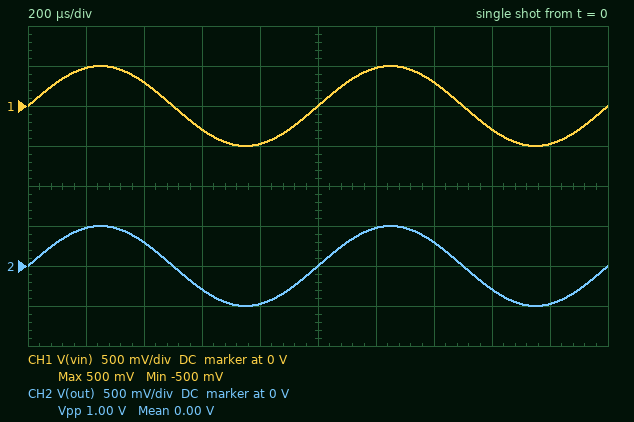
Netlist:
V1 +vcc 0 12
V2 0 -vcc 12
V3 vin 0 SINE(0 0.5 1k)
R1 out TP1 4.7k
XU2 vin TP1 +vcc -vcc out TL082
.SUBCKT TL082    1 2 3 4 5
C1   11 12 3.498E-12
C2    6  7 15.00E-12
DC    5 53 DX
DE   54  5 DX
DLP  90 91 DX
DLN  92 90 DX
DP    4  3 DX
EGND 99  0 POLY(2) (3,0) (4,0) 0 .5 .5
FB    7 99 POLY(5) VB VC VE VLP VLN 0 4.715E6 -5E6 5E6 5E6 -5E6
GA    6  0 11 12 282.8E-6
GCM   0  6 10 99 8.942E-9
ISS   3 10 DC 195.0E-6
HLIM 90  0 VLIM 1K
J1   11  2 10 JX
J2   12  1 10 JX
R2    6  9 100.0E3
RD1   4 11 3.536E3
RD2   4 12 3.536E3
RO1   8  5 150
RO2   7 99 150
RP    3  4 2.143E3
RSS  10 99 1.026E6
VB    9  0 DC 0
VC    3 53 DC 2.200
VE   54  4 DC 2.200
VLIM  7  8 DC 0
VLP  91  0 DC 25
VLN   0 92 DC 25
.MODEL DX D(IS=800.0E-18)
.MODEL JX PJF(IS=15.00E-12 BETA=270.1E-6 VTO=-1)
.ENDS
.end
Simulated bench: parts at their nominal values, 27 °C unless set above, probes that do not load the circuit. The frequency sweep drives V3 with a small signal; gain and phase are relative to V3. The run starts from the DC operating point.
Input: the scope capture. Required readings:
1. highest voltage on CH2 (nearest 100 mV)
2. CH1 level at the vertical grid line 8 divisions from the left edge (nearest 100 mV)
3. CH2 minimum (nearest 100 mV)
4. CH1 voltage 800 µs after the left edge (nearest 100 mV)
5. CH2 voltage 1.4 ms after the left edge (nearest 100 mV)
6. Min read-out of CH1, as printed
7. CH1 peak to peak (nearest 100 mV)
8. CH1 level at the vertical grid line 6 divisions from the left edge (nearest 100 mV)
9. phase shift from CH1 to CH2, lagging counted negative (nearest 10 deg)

500 mV
-300 mV
-500 mV
-500 mV
300 mV
-500 mV
1.0 V
500 mV
0 deg
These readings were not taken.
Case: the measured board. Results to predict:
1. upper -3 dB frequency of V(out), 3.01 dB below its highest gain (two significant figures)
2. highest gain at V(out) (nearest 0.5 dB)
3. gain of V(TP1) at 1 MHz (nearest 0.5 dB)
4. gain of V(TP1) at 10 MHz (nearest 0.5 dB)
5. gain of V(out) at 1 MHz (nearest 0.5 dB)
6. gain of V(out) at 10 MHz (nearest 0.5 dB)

4.9 MHz
0 dB
0 dB
-13.0 dB
0 dB
-13.0 dB
